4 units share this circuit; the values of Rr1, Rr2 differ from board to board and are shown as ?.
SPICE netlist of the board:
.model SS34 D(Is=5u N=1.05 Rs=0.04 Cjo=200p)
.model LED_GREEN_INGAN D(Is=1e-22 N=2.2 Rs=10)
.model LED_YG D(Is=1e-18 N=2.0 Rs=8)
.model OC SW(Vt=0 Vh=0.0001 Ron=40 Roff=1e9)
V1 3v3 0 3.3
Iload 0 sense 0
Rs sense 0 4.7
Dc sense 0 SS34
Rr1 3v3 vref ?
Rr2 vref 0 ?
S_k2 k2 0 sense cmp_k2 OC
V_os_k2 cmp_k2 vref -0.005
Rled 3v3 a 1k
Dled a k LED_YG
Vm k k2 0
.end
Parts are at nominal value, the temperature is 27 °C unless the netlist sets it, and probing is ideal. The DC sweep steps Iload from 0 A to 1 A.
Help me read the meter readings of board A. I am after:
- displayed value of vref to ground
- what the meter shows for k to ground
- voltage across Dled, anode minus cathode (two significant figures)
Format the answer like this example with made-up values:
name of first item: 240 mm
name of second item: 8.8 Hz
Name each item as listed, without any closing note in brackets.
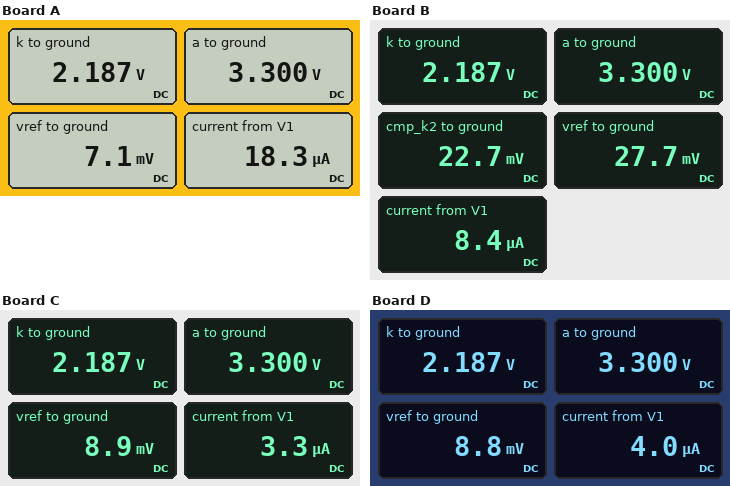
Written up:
displayed value of vref to ground: 7.1 mV
what the meter shows for k to ground: 2.187 V
voltage across Dled, anode minus cathode: 1.1 V
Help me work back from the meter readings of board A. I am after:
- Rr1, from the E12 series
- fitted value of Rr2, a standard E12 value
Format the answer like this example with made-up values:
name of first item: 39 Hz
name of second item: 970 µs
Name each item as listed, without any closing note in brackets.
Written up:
Rr1, from the E12 series: 180 kΩ
fitted value of Rr2, a standard E12 value: 390 Ω
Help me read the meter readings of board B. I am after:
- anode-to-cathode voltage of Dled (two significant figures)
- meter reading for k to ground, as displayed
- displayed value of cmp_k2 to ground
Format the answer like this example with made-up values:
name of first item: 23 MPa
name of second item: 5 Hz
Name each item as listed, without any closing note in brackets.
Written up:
anode-to-cathode voltage of Dled: 1.1 V
meter reading for k to ground, as displayed: 2.187 V
displayed value of cmp_k2 to ground: 22.7 mV
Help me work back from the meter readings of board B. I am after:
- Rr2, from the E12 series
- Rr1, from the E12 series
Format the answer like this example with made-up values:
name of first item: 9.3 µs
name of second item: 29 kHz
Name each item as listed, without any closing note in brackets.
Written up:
Rr2, from the E12 series: 3.3 kΩ
Rr1, from the E12 series: 390 kΩ
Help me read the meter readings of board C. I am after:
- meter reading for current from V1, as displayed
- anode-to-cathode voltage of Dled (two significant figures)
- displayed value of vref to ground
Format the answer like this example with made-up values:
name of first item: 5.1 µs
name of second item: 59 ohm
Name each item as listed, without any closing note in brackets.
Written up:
meter reading for current from V1, as displayed: 3.3 µA
anode-to-cathode voltage of Dled: 1.1 V
displayed value of vref to ground: 8.9 mV
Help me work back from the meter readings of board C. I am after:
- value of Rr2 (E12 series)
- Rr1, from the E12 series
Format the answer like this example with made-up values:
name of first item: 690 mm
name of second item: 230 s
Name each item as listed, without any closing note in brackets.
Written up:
value of Rr2: 2.7 kΩ
Rr1, from the E12 series: 1 MΩ
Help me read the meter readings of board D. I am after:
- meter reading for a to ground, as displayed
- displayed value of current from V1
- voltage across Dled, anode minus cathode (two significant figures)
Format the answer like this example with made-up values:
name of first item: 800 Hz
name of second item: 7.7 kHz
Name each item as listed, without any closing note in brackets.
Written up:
meter reading for a to ground, as displayed: 3.300 V
displayed value of current from V1: 4.0 µA
voltage across Dled, anode minus cathode: 1.1 V
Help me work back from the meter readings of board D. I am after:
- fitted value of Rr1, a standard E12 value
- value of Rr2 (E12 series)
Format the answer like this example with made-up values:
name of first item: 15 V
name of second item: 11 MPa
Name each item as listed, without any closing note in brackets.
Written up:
fitted value of Rr1, a standard E12 value: 820 kΩ
value of Rr2: 2.2 kΩ
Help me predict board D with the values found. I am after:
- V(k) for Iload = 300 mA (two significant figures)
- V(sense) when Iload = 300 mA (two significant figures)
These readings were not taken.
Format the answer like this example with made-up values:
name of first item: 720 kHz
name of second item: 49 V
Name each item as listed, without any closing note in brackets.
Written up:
V(k) for Iload = 300 mA: 57 mV
V(sense) when Iload = 300 mA: 300 mV
